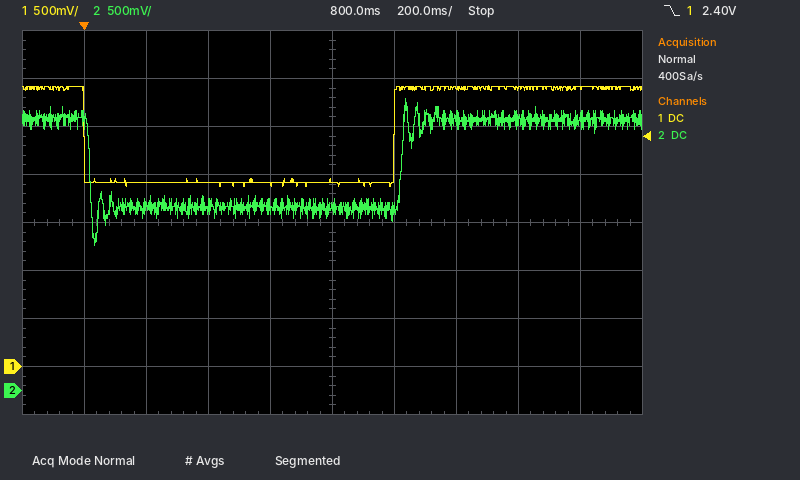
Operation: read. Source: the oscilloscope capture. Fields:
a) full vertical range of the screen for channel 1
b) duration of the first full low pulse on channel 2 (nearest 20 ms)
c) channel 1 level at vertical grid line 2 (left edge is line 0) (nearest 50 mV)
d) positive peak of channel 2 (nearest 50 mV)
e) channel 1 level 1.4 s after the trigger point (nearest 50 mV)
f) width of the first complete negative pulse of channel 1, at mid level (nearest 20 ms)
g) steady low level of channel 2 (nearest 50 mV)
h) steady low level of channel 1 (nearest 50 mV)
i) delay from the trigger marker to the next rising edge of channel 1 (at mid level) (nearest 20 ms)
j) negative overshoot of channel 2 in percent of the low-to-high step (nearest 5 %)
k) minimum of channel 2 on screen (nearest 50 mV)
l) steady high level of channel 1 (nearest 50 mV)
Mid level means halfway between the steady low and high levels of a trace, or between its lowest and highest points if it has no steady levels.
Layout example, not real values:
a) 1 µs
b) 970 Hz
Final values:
a) 4 V
b) 1.00 s
c) 1.90 V
d) 3.05 V
e) 2.90 V
f) 1.00 s
g) 1.90 V
h) 1.90 V
i) 1.00 s
j) 45 %
k) 1.50 V
l) 2.90 V
